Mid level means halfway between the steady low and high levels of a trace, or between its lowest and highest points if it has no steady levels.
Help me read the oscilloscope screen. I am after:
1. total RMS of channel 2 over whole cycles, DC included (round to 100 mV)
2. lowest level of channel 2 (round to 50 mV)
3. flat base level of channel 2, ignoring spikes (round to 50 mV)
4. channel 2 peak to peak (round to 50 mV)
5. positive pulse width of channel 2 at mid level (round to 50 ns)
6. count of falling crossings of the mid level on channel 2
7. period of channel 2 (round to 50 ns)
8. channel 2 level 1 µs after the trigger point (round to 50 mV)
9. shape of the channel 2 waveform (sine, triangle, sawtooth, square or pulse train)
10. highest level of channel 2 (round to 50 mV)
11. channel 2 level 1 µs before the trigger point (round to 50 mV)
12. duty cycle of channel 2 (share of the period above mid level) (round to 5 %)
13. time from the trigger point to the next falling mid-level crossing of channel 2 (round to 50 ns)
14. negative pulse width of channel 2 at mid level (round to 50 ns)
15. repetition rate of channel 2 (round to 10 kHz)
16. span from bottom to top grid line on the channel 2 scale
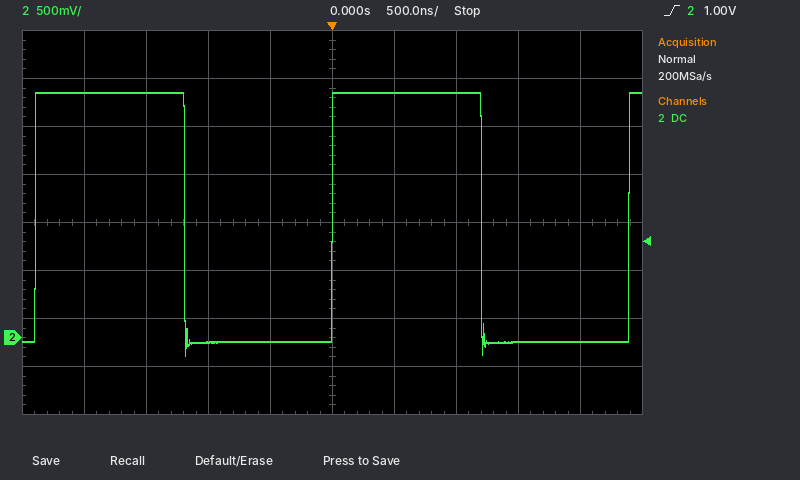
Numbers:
1.8 V
-200 mV
-50 mV
2.75 V
1.20 µs
2
2.40 µs
2.55 V
square
2.55 V
-50 mV
50 %
1.20 µs
1.20 µs
420 kHz
4 V
